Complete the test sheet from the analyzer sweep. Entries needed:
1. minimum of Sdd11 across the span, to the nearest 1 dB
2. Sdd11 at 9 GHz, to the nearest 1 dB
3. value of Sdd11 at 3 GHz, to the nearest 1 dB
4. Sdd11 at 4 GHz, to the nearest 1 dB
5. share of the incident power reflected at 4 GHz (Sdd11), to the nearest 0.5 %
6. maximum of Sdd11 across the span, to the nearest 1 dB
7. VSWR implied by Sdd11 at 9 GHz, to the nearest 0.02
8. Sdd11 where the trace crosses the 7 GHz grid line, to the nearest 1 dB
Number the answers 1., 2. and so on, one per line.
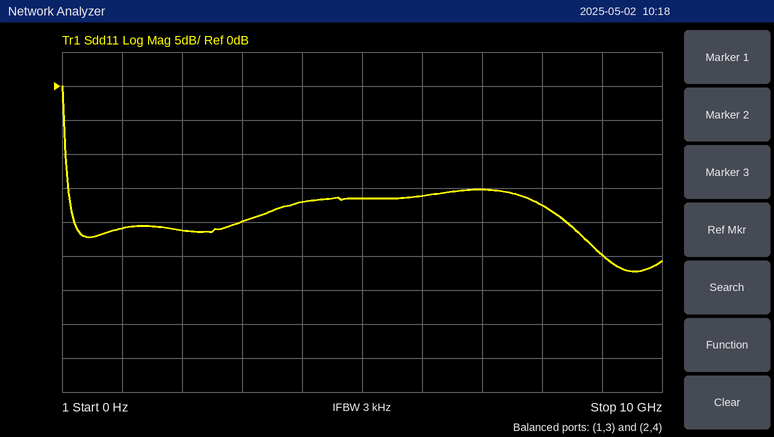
1. -27 dB
2. -25 dB
3. -20 dB
4. -17 dB
5. 2.0 %
6. 0 dB
7. 1.12
8. -15 dB
